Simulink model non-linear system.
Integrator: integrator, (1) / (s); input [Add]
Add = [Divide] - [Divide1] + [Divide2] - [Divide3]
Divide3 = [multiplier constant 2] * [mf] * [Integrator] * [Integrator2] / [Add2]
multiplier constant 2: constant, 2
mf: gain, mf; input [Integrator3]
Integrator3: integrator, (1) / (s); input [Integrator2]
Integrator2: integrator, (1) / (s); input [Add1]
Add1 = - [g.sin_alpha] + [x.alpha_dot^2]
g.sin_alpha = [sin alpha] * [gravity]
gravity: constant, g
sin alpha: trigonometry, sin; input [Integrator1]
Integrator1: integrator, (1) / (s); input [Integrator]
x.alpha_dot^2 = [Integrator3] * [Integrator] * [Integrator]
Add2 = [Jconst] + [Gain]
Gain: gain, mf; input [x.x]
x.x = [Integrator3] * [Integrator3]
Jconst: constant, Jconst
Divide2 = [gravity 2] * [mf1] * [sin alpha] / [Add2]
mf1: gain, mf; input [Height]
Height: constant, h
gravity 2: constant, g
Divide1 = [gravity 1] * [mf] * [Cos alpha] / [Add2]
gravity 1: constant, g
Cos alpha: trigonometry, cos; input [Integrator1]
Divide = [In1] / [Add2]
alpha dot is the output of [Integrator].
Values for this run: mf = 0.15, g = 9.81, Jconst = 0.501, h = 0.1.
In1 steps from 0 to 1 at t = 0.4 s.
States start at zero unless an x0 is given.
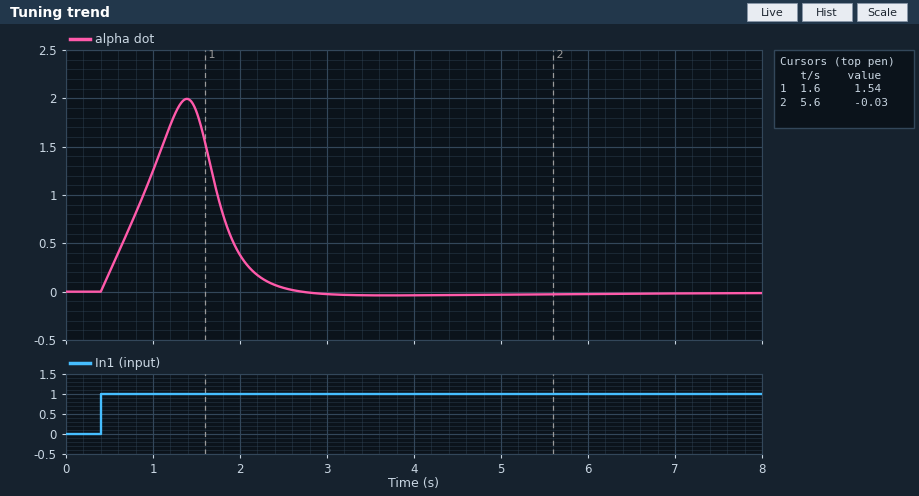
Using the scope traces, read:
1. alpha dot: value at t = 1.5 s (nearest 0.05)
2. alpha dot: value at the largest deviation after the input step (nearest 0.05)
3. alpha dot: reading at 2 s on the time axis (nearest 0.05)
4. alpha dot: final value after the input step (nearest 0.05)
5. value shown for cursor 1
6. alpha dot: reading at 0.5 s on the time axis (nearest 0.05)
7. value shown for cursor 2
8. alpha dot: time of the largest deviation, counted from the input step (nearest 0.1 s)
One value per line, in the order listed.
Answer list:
1.85
2.00
0.40
0.00
1.54
0.20
-0.03
1.0 s
